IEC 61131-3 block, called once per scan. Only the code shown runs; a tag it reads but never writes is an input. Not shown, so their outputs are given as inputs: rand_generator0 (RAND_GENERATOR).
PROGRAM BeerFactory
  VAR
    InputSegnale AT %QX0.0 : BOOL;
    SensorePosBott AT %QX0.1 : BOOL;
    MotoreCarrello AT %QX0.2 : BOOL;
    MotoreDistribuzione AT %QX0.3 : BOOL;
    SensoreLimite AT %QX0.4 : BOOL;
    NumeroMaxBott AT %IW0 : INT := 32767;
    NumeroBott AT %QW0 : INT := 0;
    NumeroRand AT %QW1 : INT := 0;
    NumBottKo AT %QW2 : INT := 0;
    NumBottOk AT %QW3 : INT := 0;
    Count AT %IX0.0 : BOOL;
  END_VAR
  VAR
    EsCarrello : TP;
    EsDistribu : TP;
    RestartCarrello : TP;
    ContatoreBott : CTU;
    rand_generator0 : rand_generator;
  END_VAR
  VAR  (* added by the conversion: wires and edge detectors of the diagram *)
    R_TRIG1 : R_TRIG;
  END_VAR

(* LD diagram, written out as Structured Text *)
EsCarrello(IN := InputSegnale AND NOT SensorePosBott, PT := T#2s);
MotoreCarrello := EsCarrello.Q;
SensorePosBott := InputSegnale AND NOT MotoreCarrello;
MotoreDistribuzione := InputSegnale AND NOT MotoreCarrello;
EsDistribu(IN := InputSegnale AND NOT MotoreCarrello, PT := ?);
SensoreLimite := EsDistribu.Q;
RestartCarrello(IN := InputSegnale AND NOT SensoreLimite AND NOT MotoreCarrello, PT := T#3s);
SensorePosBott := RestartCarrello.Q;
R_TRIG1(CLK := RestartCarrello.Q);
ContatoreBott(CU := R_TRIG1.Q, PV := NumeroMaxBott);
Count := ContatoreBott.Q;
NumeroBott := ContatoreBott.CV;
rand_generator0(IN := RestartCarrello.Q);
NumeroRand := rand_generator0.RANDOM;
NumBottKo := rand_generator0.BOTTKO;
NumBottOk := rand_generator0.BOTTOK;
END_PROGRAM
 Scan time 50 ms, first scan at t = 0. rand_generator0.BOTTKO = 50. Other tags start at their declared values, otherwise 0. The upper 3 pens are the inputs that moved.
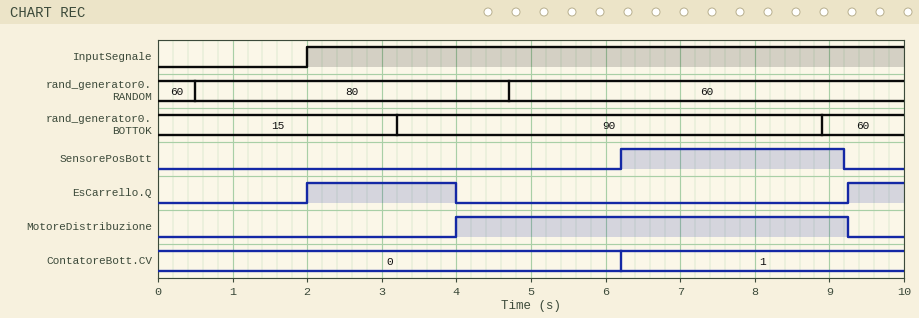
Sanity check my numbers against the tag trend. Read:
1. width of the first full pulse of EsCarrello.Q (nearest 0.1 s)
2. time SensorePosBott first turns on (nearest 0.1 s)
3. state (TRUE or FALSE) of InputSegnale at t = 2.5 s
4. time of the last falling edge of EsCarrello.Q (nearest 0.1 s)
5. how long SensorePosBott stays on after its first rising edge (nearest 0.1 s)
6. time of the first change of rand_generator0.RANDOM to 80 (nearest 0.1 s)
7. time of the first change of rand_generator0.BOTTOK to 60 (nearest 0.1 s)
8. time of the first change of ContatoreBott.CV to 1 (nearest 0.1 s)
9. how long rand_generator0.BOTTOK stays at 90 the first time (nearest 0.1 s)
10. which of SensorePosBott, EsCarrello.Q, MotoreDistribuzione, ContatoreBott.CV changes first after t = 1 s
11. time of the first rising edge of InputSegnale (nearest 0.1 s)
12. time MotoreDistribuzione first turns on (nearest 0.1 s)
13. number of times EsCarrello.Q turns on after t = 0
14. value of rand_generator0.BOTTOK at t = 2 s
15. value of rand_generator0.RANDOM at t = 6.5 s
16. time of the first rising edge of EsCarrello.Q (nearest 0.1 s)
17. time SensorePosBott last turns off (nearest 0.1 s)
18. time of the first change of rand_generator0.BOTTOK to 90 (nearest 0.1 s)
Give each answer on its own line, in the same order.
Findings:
2.0 s
6.2 s
TRUE
4.0 s
3.0 s
0.5 s
8.9 s
6.2 s
5.7 s
EsCarrello.Q
2.0 s
4.0 s
2
15
60
2.0 s
9.2 s
3.2 s
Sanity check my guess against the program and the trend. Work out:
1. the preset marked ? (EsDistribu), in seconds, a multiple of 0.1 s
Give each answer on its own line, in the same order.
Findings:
2.2 s
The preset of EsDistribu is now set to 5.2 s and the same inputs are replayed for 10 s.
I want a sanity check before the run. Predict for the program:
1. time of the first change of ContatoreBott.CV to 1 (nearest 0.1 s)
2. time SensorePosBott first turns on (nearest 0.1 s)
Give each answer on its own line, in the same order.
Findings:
9.2 s
9.2 s
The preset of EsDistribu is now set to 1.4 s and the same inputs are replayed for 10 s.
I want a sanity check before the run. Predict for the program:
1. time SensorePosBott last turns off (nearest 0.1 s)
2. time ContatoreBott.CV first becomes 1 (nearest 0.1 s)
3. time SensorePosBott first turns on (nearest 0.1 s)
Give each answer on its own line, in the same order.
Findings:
8.4 s
5.4 s
5.4 s
